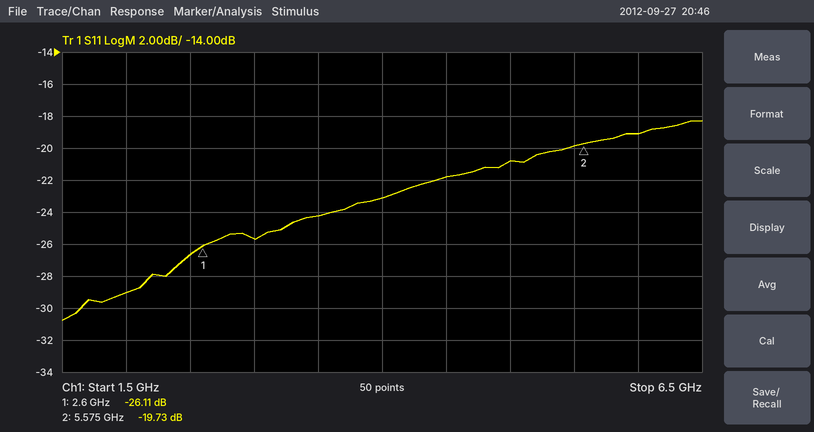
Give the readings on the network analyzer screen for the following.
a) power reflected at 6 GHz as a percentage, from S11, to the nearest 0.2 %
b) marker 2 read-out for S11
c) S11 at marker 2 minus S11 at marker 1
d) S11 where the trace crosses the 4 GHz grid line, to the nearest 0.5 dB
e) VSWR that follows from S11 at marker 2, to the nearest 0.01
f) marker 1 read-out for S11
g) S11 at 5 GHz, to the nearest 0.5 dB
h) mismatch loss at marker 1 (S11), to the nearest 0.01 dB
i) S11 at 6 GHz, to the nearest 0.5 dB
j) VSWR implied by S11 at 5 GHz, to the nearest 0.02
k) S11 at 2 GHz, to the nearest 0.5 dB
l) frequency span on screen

1.2 %
-19.73 dB
6.38 dB
-23.0 dB
1.23
-26.11 dB
-21.0 dB
0.01 dB
-19.0 dB
1.20
-29.0 dB
5 GHz
